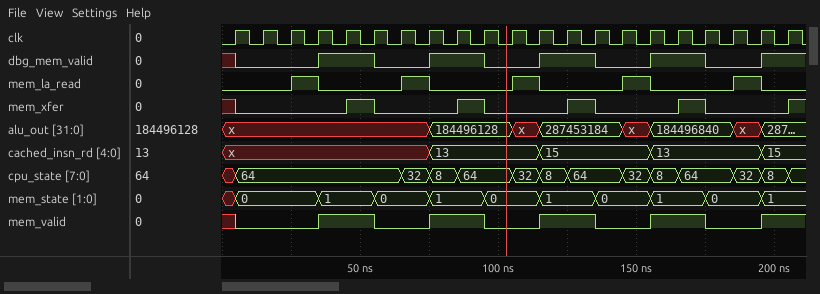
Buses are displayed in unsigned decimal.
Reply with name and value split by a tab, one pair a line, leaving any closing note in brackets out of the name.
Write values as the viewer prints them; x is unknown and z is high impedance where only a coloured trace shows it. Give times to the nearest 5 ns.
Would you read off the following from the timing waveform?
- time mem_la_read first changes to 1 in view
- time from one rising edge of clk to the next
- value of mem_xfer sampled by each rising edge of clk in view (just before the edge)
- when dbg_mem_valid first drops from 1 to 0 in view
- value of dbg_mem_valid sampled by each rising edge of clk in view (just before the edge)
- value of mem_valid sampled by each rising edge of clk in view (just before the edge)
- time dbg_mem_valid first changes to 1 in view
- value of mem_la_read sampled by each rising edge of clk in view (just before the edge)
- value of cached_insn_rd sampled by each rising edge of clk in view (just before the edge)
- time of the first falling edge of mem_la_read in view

time mem_la_read first changes to 1 in view	25 ns
time from one rising edge of clk to the next	10 ns
value of mem_xfer sampled by each rising edge of clk in view	x 0 0 0 0 1 0 0 0 1 0 0 0 1 0 0 0 1 0 0 0
when dbg_mem_valid first drops from 1 to 0 in view	55 ns
value of dbg_mem_valid sampled by each rising edge of clk in view	x 0 0 0 1 1 0 0 1 1 0 0 1 1 0 0 1 1 0 0 1
value of mem_valid sampled by each rising edge of clk in view	x 0 0 0 1 1 0 0 1 1 0 0 1 1 0 0 1 1 0 0 1
time dbg_mem_valid first changes to 1 in view	35 ns
value of mem_la_read sampled by each rising edge of clk in view	0 0 0 1 0 0 0 1 0 0 0 1 0 0 0 1 0 0 0 1 0
value of cached_insn_rd sampled by each rising edge of clk in view	x, x, x, x, x, x, x, x, 13, 13, 13, 13, 15, 15, 15, 15, 13, 13, 13, 13, 15
time of the first falling edge of mem_la_read in view	35 ns
